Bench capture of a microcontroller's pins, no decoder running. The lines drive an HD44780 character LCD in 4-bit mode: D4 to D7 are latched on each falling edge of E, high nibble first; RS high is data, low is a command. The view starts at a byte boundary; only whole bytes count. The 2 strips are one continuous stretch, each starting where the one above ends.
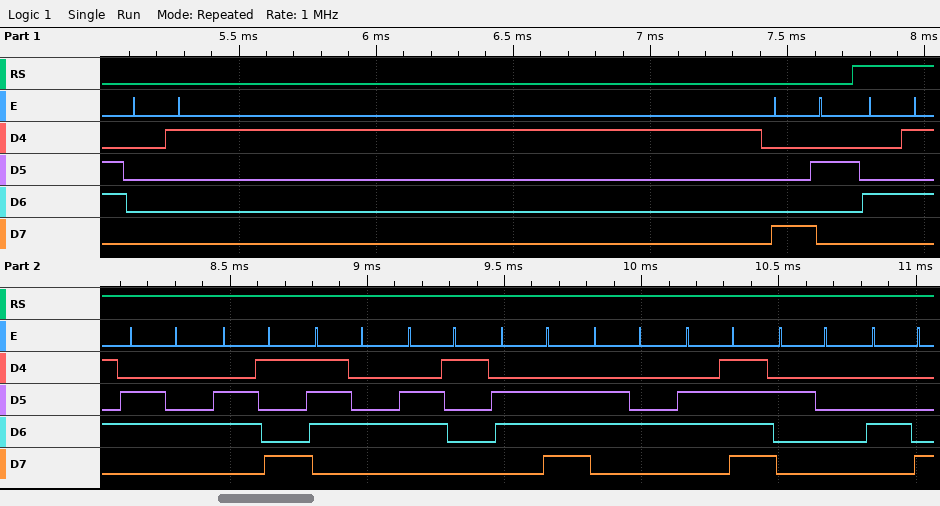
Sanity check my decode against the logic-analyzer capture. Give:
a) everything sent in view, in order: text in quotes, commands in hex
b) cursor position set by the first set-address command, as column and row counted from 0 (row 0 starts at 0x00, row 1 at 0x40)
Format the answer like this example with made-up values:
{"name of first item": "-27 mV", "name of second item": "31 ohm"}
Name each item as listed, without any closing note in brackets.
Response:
{"everything sent in view, in order: text in quotes, commands in hex": "0x01 0x82 \"Editando H\"", "cursor position set by the first set-address command, as column and row counted from 0": "column 2, row 0"}
